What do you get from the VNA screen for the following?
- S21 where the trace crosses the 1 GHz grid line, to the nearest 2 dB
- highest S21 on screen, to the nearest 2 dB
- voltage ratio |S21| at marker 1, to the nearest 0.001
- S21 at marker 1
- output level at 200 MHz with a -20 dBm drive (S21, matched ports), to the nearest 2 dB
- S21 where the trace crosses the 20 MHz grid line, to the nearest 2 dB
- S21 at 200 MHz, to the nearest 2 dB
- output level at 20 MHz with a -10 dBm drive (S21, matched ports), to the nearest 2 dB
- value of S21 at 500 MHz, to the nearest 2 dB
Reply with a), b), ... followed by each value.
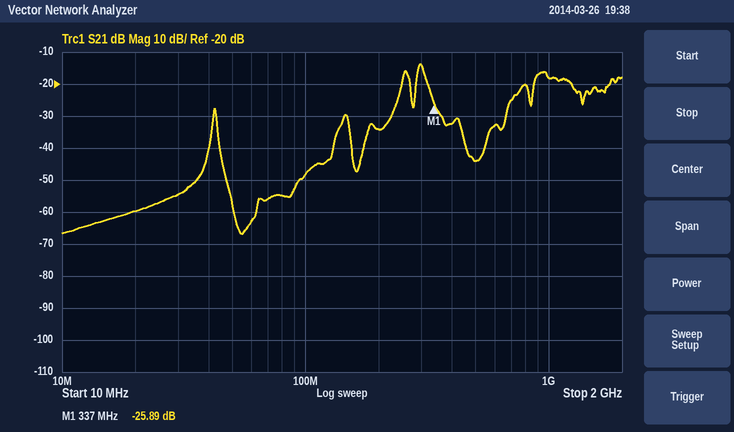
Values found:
a) -18 dB
b) -14 dB
c) 0.051
d) -25.89 dB
e) -54 dBm
f) -60 dB
g) -34 dB
h) -70 dBm
i) -44 dB
